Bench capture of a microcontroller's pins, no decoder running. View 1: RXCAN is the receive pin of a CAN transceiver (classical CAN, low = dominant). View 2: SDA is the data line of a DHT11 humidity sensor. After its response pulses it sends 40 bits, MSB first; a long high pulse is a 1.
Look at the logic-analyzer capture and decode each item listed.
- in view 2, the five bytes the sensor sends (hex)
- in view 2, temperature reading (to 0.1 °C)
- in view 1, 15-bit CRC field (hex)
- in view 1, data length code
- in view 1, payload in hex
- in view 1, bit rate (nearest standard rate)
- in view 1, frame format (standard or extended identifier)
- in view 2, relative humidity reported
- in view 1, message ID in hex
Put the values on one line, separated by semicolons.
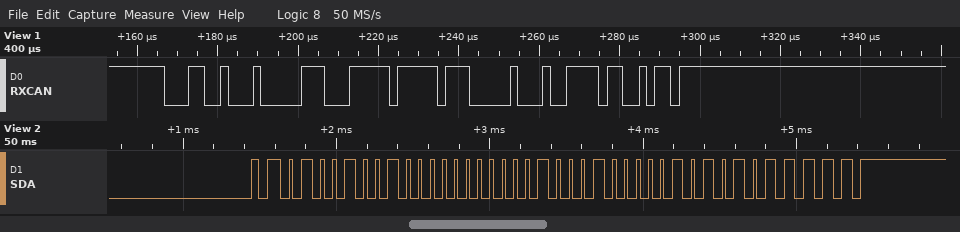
49 00 11 05 5F; 17.5 °C; 0x4F65; 3; 1F FF 00; 500 kbit/s; standard; 73 %; 0x191
